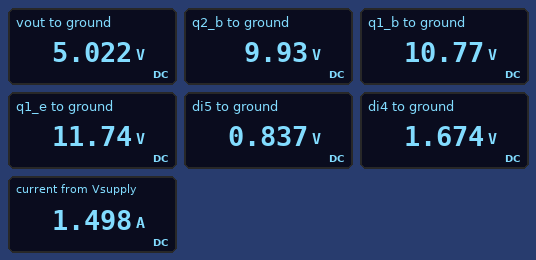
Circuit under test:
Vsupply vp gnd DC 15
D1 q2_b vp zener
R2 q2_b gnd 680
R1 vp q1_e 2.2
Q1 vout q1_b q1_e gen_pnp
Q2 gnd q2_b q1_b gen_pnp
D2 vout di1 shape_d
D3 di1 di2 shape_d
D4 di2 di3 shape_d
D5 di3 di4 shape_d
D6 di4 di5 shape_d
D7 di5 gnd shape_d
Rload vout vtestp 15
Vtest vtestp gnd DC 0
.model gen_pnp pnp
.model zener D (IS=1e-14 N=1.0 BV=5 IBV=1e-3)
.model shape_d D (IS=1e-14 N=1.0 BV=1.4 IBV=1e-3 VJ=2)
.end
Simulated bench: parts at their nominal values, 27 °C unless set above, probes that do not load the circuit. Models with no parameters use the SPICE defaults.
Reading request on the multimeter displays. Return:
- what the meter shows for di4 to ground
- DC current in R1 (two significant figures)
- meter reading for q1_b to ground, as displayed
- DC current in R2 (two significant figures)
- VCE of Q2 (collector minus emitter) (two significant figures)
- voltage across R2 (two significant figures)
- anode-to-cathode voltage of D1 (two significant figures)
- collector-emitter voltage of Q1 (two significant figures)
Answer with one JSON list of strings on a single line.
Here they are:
["1.674 V", "1.5 A", "10.77 V", "15 mA", "-11 V", "9.9 V", "-5.1 V", "-6.7 V"]
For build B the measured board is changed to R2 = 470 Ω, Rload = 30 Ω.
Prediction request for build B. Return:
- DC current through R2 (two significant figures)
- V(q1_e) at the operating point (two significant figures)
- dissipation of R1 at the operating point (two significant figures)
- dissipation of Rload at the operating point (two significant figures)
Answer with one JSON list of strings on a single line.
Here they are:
["21 mA", "12 V", "4.9 W", "850 mW"]
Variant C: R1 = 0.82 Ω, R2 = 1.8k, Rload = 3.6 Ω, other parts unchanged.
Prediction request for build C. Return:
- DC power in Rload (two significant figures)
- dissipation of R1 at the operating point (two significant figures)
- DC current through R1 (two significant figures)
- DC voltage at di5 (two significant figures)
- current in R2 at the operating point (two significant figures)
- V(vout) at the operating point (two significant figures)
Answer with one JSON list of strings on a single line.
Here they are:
["7.3 W", "12 W", "3.9 A", "860 mV", "5.5 mA", "5.1 V"]
